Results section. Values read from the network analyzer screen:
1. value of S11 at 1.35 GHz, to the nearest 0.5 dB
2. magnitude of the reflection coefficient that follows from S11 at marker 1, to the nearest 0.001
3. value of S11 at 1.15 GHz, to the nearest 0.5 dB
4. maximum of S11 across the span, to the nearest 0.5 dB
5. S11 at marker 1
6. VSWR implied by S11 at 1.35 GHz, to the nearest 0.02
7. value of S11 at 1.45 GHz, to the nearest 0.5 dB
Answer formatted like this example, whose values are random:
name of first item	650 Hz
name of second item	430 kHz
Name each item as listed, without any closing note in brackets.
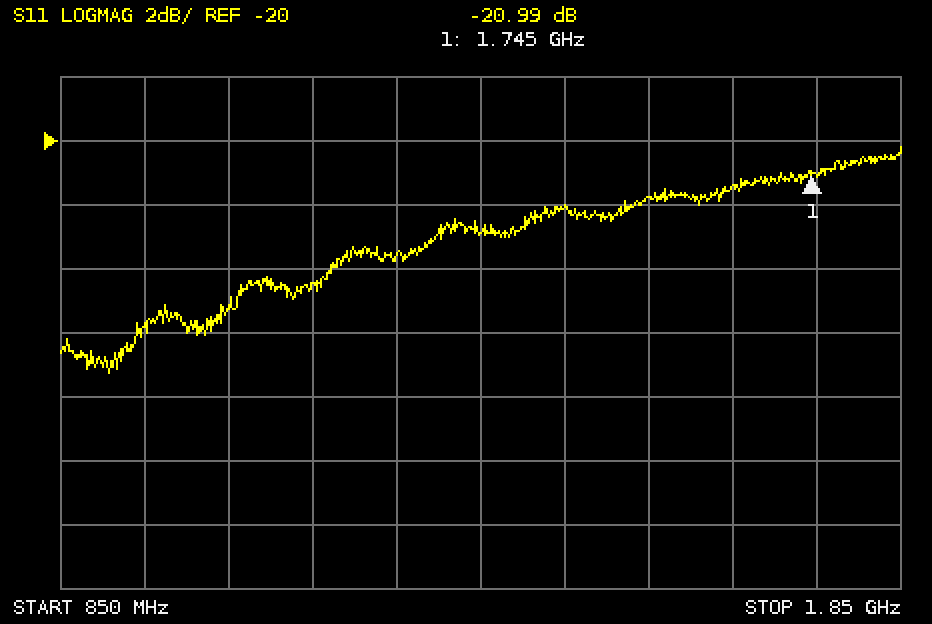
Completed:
value of S11 at 1.35 GHz, to the nearest 0.5 dB	-23.0 dB
magnitude of the reflection coefficient that follows from S11 at marker 1, to the nearest 0.001	0.089
value of S11 at 1.15 GHz, to the nearest 0.5 dB	-24.5 dB
maximum of S11 across the span, to the nearest 0.5 dB	-20.0 dB
S11 at marker 1	-20.99 dB
VSWR implied by S11 at 1.35 GHz, to the nearest 0.02	1.16
value of S11 at 1.45 GHz, to the nearest 0.5 dB	-22.0 dB
